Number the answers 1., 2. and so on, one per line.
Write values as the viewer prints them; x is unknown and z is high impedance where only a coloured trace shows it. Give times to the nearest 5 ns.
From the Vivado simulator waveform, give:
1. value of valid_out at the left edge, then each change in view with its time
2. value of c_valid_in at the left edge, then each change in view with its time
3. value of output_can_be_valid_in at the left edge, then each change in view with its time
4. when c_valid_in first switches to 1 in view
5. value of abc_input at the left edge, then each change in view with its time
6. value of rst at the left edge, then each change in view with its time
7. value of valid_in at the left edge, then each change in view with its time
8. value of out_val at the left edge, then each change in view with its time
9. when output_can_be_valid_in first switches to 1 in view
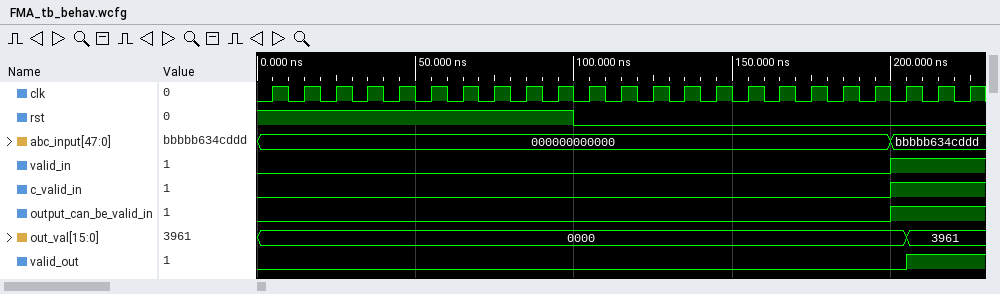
1. 0, 1 at 205 ns
2. 0, 1 at 200 ns
3. 0, 1 at 200 ns
4. 200 ns
5. 000000000000, bbbbb634cddd at 200 ns
6. 1, 0 at 100 ns
7. 0, 1 at 200 ns
8. 0000, 3961 at 205 ns
9. 200 ns
